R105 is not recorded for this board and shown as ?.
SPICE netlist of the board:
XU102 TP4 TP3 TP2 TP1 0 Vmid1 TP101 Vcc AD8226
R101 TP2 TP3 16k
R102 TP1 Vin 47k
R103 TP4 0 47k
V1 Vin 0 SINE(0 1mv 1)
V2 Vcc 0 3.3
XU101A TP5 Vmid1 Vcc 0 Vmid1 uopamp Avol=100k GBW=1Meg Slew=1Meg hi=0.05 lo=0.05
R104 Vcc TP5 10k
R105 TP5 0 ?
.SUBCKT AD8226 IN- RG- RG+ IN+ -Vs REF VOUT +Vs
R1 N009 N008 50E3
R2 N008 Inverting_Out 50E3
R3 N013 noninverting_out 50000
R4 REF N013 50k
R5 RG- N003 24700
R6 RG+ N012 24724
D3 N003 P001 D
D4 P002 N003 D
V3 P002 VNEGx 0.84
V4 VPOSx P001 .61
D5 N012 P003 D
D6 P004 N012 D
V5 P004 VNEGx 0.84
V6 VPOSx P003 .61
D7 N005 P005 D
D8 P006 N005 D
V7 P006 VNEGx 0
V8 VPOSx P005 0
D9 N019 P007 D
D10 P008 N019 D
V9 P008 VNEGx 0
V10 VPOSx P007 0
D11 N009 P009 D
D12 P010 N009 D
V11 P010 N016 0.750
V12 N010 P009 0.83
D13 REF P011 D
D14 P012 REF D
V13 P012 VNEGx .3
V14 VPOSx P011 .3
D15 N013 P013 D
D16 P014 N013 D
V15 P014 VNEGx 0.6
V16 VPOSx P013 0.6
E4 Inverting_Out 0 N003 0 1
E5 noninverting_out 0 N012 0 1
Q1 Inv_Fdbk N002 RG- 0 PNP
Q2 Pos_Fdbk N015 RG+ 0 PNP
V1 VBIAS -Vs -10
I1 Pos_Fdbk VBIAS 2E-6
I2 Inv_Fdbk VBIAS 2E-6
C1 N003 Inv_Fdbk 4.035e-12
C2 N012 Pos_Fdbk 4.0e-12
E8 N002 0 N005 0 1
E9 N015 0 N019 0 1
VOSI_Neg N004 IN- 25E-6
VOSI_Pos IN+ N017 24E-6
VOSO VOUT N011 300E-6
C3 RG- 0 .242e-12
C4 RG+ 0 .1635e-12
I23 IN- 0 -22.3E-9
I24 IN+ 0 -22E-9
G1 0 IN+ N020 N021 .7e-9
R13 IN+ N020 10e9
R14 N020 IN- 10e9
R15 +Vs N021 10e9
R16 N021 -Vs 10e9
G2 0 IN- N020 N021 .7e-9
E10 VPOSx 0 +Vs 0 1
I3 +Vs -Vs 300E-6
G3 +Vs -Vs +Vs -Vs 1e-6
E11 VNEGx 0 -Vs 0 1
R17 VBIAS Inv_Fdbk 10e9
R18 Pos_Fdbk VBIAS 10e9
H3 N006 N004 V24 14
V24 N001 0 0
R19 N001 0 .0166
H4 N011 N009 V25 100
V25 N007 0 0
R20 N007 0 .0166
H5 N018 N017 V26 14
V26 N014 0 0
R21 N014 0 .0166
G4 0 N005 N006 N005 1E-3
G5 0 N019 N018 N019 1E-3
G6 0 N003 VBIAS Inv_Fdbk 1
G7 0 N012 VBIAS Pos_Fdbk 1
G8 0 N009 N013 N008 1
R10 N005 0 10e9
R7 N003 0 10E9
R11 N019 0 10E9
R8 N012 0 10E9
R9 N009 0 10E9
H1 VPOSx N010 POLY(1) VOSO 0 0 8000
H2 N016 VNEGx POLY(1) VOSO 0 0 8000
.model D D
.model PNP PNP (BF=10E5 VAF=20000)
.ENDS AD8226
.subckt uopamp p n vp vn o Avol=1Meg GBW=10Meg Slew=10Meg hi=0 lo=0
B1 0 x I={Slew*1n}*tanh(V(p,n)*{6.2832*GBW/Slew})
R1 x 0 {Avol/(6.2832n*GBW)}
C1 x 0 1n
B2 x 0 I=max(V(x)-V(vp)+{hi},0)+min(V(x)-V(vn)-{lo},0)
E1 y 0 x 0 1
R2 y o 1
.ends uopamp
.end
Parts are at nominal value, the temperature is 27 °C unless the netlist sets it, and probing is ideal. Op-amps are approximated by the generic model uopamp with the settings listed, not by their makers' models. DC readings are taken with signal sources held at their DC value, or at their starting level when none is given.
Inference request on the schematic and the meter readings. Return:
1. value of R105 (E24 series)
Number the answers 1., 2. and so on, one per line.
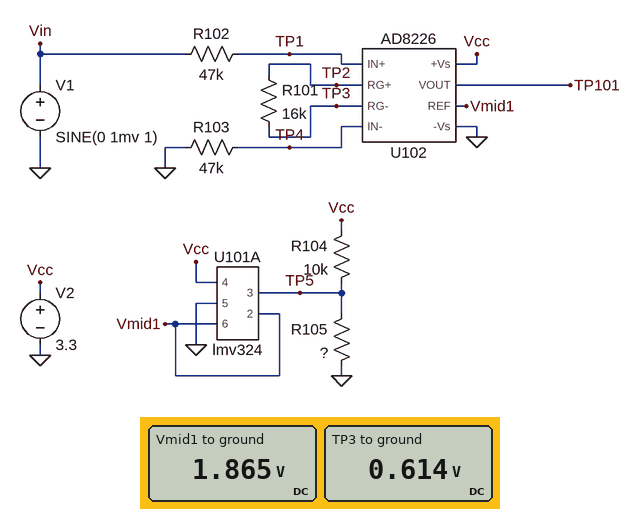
1. 13 kΩ
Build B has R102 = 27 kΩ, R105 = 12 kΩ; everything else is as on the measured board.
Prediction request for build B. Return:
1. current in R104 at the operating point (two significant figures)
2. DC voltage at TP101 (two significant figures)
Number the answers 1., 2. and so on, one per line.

1. 150 µA
2. 1.8 V
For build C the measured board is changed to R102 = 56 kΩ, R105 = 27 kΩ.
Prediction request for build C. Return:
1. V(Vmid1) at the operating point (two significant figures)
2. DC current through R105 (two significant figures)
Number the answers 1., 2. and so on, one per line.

1. 2.4 V
2. 89 µA
